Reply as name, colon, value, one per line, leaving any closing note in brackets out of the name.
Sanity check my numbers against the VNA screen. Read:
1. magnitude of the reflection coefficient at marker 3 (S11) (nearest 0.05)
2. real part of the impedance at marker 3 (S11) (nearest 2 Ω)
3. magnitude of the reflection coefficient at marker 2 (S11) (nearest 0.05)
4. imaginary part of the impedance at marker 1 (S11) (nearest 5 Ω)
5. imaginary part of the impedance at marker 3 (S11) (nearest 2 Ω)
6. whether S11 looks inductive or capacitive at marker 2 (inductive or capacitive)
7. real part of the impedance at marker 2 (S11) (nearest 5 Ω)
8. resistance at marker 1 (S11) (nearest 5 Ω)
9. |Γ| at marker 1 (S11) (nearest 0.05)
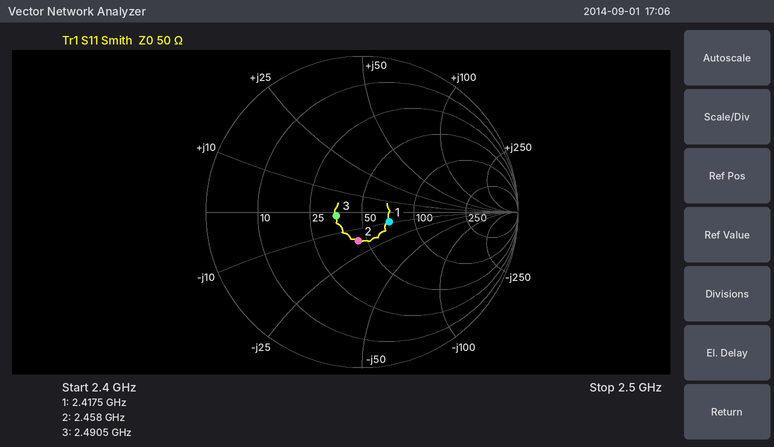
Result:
magnitude of the reflection coefficient at marker 3 (S11): 0.15
real part of the impedance at marker 3 (S11): 36 Ω
magnitude of the reflection coefficient at marker 2 (S11): 0.20
imaginary part of the impedance at marker 1 (S11): -10 Ω
imaginary part of the impedance at marker 3 (S11): -2 Ω
whether S11 looks inductive or capacitive at marker 2: capacitive
real part of the impedance at marker 2 (S11): 45 Ω
resistance at marker 1 (S11): 70 Ω
|Γ| at marker 1 (S11): 0.20
